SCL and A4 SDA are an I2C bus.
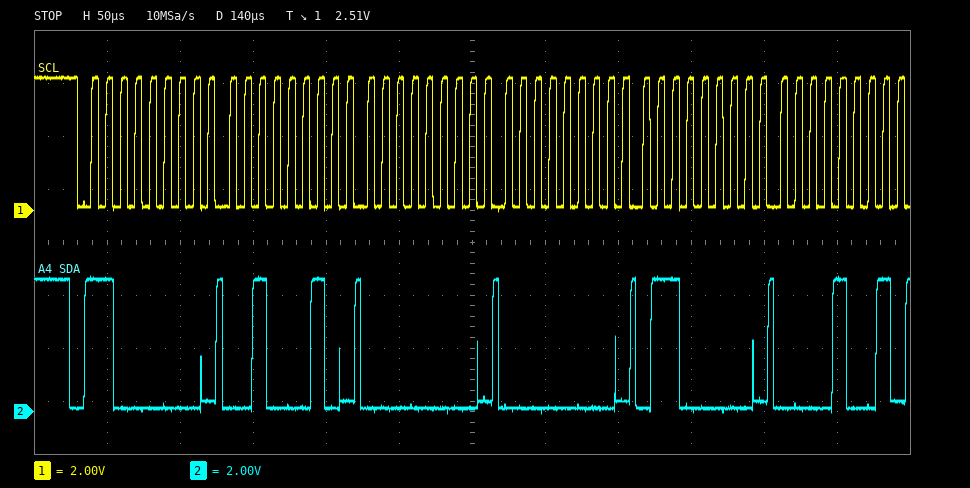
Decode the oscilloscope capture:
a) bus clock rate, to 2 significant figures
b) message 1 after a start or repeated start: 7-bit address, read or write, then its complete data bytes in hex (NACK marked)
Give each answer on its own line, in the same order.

100 kHz
0x60 write: 22 00 00 60 09
